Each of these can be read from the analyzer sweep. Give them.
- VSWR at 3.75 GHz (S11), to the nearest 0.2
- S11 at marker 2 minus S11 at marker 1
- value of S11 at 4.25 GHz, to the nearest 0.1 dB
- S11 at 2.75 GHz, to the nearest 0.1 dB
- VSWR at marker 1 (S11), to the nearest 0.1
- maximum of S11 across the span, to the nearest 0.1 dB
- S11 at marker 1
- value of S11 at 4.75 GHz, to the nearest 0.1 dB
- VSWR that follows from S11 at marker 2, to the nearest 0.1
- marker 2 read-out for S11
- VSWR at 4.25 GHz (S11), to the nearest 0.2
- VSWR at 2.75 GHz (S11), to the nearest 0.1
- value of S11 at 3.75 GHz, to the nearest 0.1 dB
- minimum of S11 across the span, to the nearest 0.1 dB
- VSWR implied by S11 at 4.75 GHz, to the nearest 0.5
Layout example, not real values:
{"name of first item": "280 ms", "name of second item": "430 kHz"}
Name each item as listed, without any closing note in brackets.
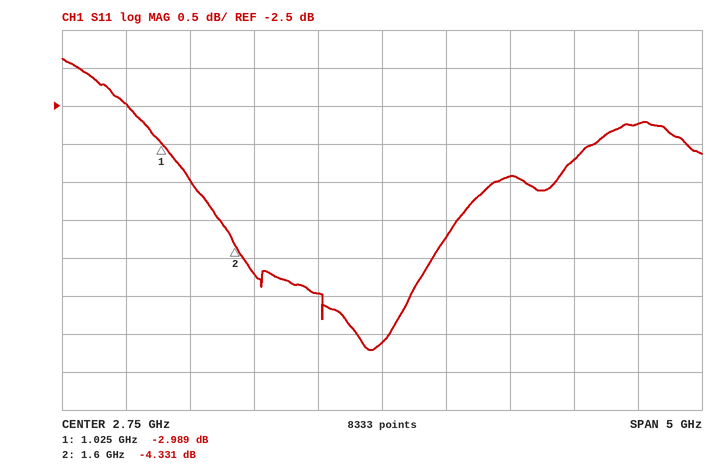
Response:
{"VSWR at 3.75 GHz (S11), to the nearest 0.2": "5.2", "S11 at marker 2 minus S11 at marker 1": "-1.342 dB", "value of S11 at 4.25 GHz, to the nearest 0.1 dB": "-3.2 dB", "S11 at 2.75 GHz, to the nearest 0.1 dB": "-5.6 dB", "VSWR at marker 1 (S11), to the nearest 0.1": "5.9", "maximum of S11 across the span, to the nearest 0.1 dB": "-1.9 dB", "S11 at marker 1": "-2.989 dB", "value of S11 at 4.75 GHz, to the nearest 0.1 dB": "-2.7 dB", "VSWR that follows from S11 at marker 2, to the nearest 0.1": "4.1", "marker 2 read-out for S11": "-4.331 dB", "VSWR at 4.25 GHz (S11), to the nearest 0.2": "5.4", "VSWR at 2.75 GHz (S11), to the nearest 0.1": "3.2", "value of S11 at 3.75 GHz, to the nearest 0.1 dB": "-3.4 dB", "minimum of S11 across the span, to the nearest 0.1 dB": "-5.7 dB", "VSWR implied by S11 at 4.75 GHz, to the nearest 0.5": "6.5"}
